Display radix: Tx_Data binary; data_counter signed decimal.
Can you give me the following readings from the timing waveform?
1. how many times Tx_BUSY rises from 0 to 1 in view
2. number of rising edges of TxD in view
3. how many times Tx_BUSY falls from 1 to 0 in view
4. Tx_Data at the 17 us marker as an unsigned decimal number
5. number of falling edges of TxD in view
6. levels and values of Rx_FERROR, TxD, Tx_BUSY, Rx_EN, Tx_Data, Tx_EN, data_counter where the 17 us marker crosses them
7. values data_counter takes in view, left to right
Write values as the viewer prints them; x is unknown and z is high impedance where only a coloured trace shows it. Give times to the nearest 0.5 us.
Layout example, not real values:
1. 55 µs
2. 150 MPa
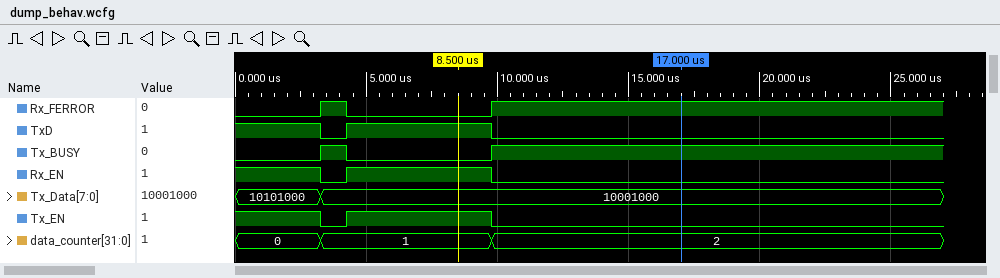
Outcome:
1. 2
2. 1
3. 1
4. 136
5. 2
6. Rx_FERROR=1, TxD=0, Tx_BUSY=1, Rx_EN=0, Tx_Data=10001000, Tx_EN=0, data_counter=2
7. 0, 1, 2
